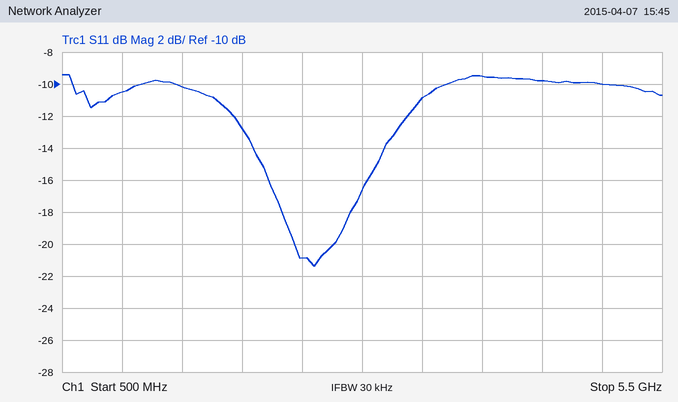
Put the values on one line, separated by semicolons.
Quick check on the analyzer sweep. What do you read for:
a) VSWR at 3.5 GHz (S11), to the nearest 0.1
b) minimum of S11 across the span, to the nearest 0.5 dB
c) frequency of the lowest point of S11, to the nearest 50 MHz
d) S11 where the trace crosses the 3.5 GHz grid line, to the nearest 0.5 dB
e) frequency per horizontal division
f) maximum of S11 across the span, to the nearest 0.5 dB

1.8; -21.5 dB; 2.60 GHz; -11.0 dB; 500 MHz; -9.5 dB
